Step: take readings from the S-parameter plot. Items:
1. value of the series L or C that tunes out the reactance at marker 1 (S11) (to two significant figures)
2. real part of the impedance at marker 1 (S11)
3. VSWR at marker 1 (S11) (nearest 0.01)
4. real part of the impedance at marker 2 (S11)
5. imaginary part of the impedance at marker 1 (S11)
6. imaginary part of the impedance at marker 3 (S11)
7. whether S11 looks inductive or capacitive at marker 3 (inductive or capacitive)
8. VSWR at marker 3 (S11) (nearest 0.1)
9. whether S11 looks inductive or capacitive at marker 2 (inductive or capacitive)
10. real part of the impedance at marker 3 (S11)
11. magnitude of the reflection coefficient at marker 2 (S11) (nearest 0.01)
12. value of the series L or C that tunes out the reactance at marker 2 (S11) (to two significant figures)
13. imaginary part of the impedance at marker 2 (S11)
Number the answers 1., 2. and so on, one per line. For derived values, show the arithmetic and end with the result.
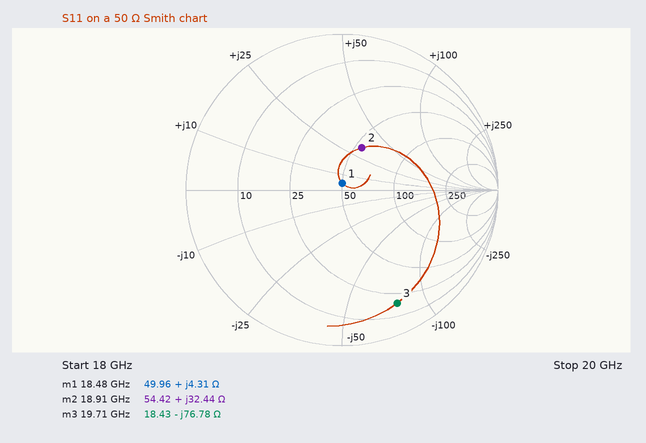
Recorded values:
1. C = 1/(2π × 18.48 GHz × 4.31 Ω) ≈ 2.0 pF
2. 49.96 Ω
3. 1.09
4. 54.42 Ω
5. +4.31 Ω
6. -76.78 Ω
7. capacitive
8. 9.4
9. inductive
10. 18.43 Ω
11. 0.30
12. C = 1/(2π × 18.91 GHz × 32.44 Ω) ≈ 259 fF, so 260 fF to two significant figures
13. +32.44 Ω
